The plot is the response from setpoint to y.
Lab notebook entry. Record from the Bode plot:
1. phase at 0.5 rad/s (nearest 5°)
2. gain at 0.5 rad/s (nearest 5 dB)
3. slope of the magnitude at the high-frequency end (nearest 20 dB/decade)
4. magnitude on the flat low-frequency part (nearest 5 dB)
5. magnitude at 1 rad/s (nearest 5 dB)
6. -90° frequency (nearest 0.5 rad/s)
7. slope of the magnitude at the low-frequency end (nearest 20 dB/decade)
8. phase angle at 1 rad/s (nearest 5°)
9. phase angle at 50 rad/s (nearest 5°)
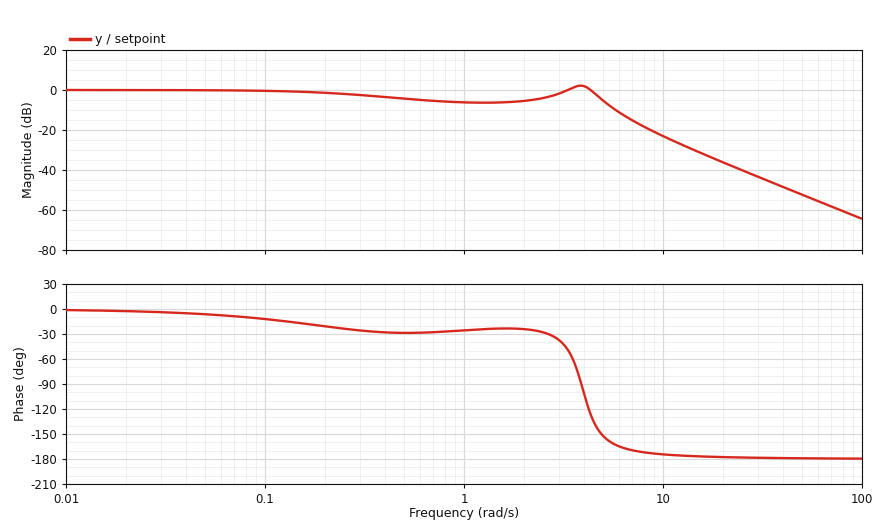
-30°
-5 dB
-40 dB/decade
0 dB
-5 dB
4.0 rad/s
0 dB/decade
-25°
-180°
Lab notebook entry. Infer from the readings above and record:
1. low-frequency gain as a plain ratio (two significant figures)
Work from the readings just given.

1.0
